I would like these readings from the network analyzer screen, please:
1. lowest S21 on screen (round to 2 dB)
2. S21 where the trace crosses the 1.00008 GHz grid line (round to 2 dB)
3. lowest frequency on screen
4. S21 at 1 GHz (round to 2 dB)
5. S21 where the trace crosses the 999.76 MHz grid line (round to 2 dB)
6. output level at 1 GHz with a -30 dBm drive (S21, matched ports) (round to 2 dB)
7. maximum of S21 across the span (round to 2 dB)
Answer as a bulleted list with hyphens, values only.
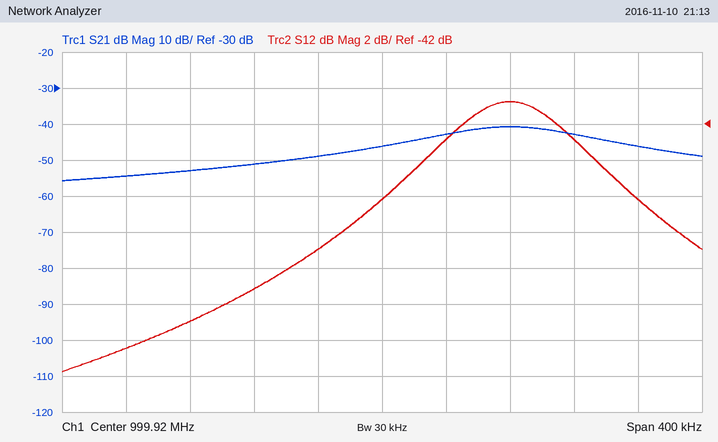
- -56 dB
- -46 dB
- 999.72 MHz
- -40 dB
- -54 dB
- -70 dBm
- -40 dB
